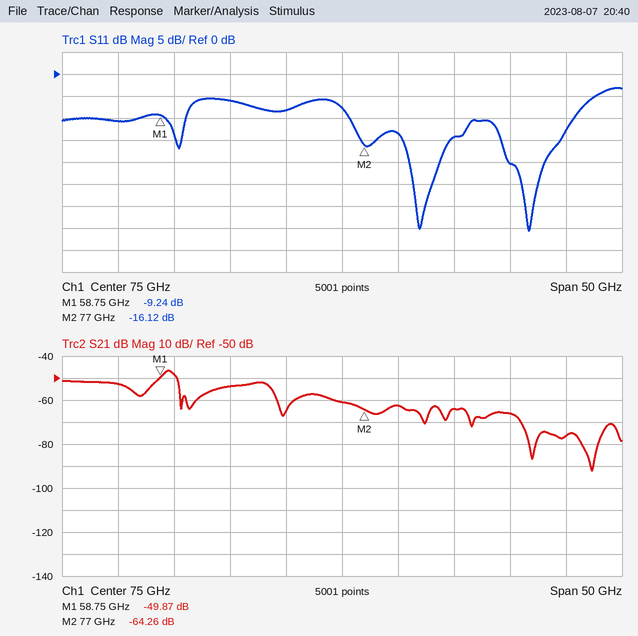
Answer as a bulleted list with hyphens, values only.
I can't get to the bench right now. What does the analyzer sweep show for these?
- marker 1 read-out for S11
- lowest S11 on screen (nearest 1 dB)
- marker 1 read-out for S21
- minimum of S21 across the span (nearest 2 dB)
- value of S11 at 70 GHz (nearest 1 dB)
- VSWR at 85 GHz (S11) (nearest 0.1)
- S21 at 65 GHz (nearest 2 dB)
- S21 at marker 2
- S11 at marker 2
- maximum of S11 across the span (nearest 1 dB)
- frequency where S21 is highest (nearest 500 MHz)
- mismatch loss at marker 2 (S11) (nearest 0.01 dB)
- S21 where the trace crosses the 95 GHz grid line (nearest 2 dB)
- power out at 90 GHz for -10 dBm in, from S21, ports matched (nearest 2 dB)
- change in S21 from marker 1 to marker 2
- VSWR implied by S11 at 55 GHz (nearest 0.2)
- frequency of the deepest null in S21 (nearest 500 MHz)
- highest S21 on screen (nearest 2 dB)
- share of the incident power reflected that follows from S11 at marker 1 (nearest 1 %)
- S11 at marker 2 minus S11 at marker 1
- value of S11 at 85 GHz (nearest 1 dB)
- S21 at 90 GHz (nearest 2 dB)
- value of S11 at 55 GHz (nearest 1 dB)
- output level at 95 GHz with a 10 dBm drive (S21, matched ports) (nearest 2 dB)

- -9.24 dB
- -36 dB
- -49.87 dB
- -92 dB
- -8 dB
- 1.5
- -54 dB
- -64.26 dB
- -16.12 dB
- -3 dB
- 59.5 GHz
- 0.11 dB
- -76 dB
- -76 dBm
- -14.39 dB
- 1.8
- 97.5 GHz
- -46 dB
- 12 %
- -6.88 dB
- -14 dB
- -66 dB
- -11 dB
- -66 dBm
